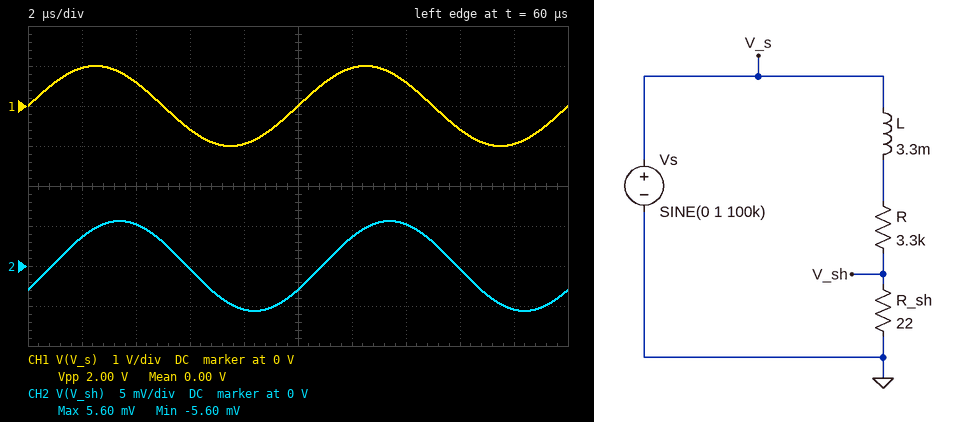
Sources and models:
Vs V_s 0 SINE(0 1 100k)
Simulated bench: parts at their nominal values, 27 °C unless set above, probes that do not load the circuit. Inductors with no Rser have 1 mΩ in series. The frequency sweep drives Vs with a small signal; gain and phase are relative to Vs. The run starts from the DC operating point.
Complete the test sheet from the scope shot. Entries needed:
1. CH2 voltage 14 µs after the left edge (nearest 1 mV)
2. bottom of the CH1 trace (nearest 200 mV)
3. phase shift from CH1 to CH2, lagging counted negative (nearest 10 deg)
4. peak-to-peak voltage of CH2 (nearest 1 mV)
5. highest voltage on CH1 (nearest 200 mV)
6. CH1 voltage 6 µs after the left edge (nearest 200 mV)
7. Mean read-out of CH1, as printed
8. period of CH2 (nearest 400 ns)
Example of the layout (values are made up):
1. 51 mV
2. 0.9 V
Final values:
1. 5 mV
2. -1.0 V
3. -30 deg
4. 11 mV
5. 1.0 V
6. -600 mV
7. 0.00 V
8. 10.0 µs
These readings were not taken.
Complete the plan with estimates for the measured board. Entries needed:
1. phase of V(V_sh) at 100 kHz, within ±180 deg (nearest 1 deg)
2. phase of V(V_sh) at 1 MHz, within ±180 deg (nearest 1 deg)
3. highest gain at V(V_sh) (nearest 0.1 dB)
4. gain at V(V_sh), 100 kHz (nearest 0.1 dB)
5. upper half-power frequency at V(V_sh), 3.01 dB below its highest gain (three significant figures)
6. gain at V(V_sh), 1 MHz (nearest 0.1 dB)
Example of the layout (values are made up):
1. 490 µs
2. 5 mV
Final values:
1. -32 deg
2. -81 deg
3. -43.6 dB
4. -45.0 dB
5. 160 kHz
6. -59.6 dB
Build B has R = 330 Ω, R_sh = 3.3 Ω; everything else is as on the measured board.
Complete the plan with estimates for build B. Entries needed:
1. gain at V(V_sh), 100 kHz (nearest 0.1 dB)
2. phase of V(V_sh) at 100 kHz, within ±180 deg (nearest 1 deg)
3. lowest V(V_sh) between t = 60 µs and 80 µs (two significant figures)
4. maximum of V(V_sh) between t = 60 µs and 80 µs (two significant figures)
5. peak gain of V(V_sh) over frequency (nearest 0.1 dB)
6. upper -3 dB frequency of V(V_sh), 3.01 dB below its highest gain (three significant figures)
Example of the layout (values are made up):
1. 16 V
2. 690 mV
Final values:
1. -56.1 dB
2. -81 deg
3. -1.6 mV
4. 1.6 mV
5. -40.1 dB
6. 16.1 kHz
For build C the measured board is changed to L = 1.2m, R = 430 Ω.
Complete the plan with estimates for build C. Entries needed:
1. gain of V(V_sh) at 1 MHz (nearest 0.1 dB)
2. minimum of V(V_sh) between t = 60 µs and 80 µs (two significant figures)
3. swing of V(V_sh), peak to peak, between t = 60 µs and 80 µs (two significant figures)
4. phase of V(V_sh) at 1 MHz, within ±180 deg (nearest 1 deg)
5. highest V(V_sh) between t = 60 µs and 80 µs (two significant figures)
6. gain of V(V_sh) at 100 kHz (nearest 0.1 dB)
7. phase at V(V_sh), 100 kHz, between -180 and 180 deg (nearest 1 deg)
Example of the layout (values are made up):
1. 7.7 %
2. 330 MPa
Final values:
1. -50.7 dB
2. -25 mV
3. 50 mV
4. -87 deg
5. 25 mV
6. -32.0 dB
7. -59 deg
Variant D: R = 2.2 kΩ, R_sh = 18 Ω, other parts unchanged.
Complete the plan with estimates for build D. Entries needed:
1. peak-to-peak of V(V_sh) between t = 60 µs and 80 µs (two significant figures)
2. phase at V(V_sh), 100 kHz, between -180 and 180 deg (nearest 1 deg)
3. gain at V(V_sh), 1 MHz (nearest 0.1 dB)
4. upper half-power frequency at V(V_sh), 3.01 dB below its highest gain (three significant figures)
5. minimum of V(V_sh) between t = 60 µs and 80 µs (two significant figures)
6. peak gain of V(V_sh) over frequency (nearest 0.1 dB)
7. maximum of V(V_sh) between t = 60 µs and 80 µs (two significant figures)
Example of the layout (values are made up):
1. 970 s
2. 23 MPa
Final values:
1. 12 mV
2. -43 deg
3. -61.3 dB
4. 107 kHz
5. -5.9 mV
6. -41.8 dB
7. 5.9 mV
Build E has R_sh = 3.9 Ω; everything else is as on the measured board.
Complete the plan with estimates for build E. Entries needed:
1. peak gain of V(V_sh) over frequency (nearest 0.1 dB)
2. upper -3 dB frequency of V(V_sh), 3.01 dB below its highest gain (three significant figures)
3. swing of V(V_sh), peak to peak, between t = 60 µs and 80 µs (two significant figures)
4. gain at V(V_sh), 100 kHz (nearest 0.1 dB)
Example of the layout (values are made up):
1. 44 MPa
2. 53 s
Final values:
1. -58.6 dB
2. 159 kHz
3. 2.0 mV
4. -60.0 dB
